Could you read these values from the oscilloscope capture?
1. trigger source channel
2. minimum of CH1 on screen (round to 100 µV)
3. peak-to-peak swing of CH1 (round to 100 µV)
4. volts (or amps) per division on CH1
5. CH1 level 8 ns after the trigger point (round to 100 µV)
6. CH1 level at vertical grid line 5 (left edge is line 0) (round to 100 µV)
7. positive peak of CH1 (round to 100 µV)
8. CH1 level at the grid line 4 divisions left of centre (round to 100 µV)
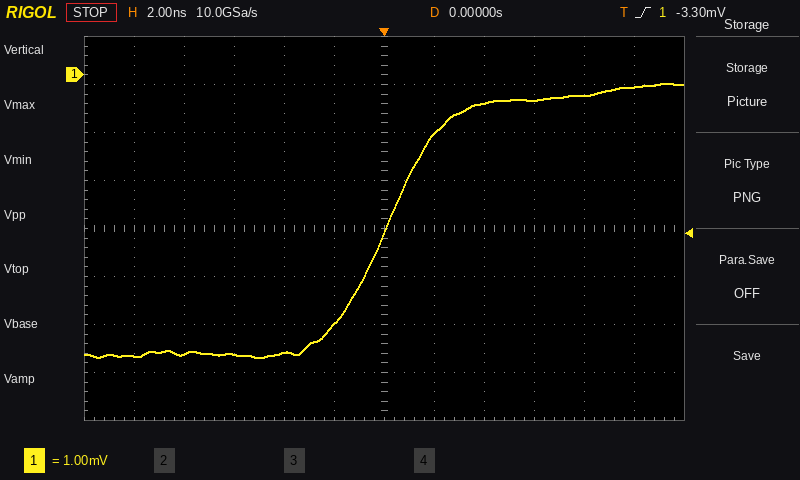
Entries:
CH1
-5.9 mV
5.7 mV
1 mV
-400 µV
-5.2 mV
-200 µV
-5.8 mV
